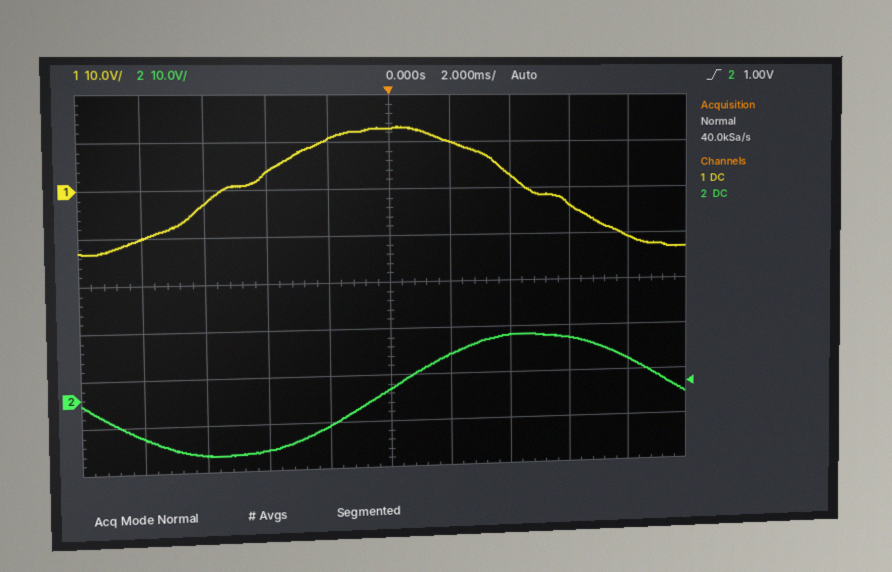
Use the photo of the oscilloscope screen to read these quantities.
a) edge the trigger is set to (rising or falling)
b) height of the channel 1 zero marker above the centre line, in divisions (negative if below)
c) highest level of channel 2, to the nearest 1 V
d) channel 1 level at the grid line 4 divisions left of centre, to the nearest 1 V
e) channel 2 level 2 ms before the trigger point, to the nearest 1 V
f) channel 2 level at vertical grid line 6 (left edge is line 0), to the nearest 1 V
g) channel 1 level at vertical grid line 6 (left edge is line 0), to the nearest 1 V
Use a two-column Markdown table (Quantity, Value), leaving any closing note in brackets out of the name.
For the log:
| Quantity | Value |
|---|---|
| edge the trigger is set to | rising |
| height of the channel 1 zero marker above the centre line, in divisions | +2.0 div |
| highest level of channel 2, to the nearest 1 V | 12 V |
| channel 1 level at the grid line 4 divisions left of centre, to the nearest 1 V | -10 V |
| channel 2 level 2 ms before the trigger point, to the nearest 1 V | -7 V |
| channel 2 level at vertical grid line 6 (left edge is line 0), to the nearest 1 V | 8 V |
| channel 1 level at vertical grid line 6 (left edge is line 0), to the nearest 1 V | 10 V |
